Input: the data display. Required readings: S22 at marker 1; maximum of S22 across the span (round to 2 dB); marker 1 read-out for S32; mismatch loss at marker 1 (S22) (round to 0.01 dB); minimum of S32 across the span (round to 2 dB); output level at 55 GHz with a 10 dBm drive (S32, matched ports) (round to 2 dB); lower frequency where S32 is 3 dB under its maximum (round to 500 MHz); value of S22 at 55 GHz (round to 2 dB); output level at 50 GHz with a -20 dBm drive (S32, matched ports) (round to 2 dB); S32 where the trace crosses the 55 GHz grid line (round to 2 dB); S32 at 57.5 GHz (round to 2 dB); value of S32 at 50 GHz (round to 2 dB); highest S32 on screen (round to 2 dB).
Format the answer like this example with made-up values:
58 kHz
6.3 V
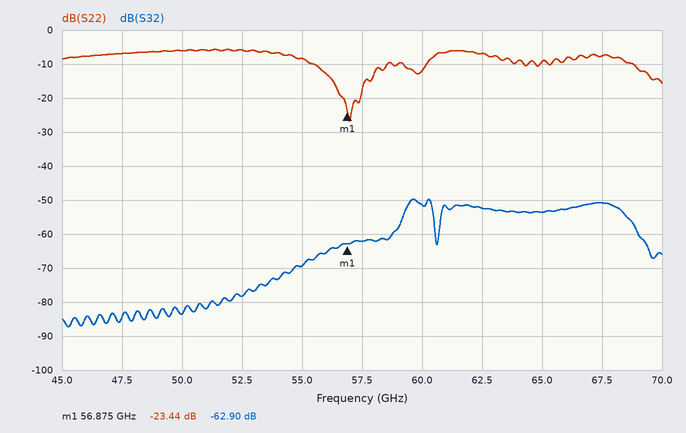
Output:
-23.44 dB
-6 dB
-62.90 dB
0.02 dB
-88 dB
-60 dBm
59.5 GHz
-8 dB
-104 dBm
-70 dB
-62 dB
-84 dB
-50 dB
